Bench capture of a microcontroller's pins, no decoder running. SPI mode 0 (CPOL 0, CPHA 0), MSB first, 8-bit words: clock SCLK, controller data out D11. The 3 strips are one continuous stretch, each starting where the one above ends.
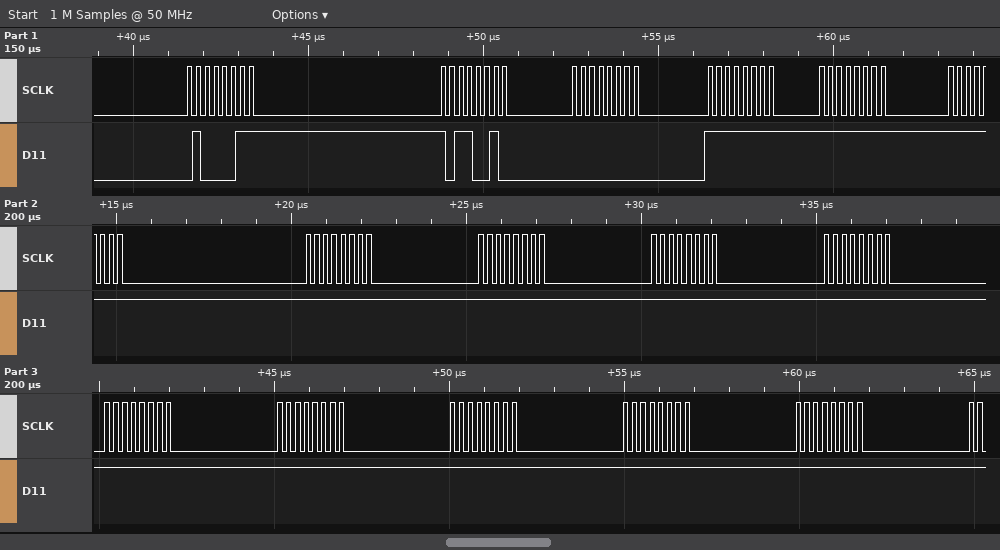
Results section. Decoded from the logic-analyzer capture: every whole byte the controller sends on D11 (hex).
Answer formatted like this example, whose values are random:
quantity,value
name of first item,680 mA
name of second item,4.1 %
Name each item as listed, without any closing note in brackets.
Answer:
quantity,value
every whole byte the controller sends on D11,43 B2 00 FF FF FF FF FF FF FF FF FF FF FF FF
